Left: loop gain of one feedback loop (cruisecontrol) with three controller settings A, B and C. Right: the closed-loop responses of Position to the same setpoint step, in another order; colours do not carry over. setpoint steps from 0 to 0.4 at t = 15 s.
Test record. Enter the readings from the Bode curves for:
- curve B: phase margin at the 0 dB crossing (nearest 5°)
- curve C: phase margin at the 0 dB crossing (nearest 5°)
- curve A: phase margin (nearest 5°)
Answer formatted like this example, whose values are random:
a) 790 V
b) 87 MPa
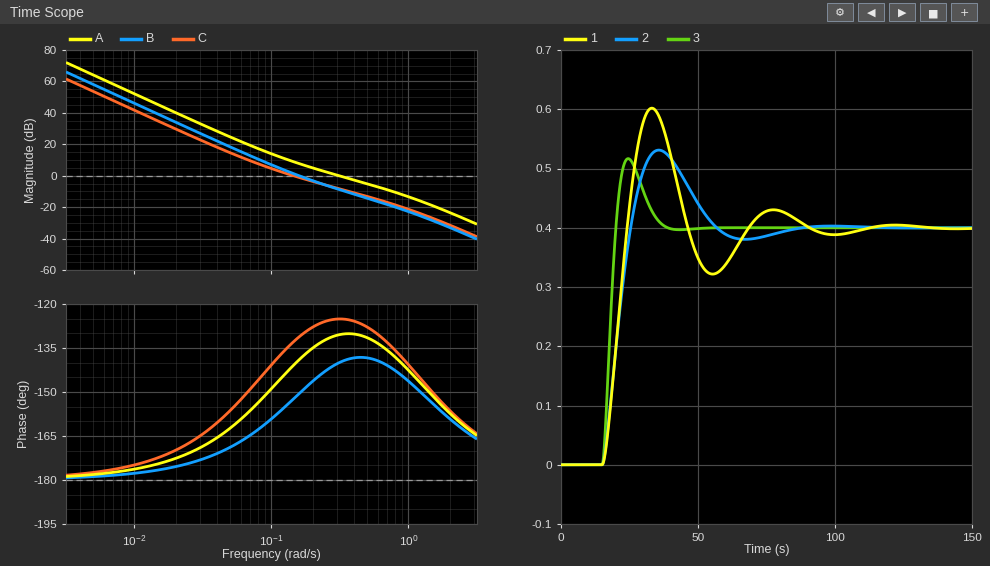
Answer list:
a) 30°
b) 45°
c) 50°
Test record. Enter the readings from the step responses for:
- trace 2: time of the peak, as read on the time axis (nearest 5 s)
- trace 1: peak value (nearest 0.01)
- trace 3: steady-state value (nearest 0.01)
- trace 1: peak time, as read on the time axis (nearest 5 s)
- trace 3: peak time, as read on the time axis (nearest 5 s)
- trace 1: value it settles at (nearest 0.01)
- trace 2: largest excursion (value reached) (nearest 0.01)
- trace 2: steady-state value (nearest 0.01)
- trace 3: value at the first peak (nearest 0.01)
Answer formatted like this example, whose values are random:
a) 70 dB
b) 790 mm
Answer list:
a) 35 s
b) 0.60
c) 0.40
d) 35 s
e) 25 s
f) 0.40
g) 0.53
h) 0.40
i) 0.52
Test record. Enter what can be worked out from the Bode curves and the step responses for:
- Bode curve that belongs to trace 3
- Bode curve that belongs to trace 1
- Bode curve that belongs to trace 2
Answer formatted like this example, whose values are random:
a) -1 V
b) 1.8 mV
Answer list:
a) A
b) B
c) C
